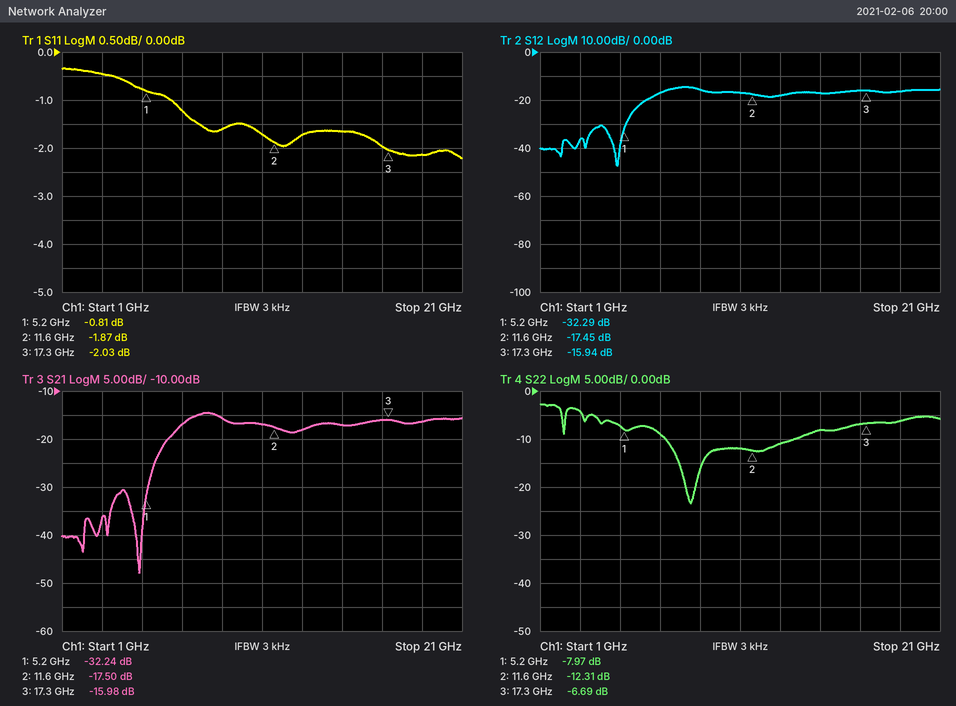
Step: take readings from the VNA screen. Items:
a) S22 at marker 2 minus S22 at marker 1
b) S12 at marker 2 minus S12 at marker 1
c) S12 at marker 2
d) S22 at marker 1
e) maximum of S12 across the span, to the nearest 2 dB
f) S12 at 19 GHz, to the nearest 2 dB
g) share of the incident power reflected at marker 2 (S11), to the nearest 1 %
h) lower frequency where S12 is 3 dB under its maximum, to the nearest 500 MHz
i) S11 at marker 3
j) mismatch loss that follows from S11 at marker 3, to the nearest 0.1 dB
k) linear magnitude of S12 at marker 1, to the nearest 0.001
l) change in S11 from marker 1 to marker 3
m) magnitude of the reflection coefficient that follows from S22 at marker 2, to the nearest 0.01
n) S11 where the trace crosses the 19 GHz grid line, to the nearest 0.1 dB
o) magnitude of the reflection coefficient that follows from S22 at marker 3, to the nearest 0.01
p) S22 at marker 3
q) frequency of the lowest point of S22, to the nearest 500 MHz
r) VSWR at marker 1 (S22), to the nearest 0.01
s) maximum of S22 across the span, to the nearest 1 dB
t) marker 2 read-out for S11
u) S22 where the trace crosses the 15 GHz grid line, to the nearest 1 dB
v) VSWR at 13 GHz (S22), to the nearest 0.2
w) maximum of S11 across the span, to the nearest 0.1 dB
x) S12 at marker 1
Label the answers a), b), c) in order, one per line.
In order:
a) -4.34 dB
b) 14.84 dB
c) -17.45 dB
d) -7.97 dB
e) -14 dB
f) -16 dB
g) 65 %
h) 7.0 GHz
i) -2.03 dB
j) 4.3 dB
k) 0.024
l) -1.22 dB
m) 0.24
n) -2.1 dB
o) 0.46
p) -6.69 dB
q) 8.5 GHz
r) 2.33
s) -3 dB
t) -1.87 dB
u) -8 dB
v) 1.8
w) -0.3 dB
x) -32.29 dB
